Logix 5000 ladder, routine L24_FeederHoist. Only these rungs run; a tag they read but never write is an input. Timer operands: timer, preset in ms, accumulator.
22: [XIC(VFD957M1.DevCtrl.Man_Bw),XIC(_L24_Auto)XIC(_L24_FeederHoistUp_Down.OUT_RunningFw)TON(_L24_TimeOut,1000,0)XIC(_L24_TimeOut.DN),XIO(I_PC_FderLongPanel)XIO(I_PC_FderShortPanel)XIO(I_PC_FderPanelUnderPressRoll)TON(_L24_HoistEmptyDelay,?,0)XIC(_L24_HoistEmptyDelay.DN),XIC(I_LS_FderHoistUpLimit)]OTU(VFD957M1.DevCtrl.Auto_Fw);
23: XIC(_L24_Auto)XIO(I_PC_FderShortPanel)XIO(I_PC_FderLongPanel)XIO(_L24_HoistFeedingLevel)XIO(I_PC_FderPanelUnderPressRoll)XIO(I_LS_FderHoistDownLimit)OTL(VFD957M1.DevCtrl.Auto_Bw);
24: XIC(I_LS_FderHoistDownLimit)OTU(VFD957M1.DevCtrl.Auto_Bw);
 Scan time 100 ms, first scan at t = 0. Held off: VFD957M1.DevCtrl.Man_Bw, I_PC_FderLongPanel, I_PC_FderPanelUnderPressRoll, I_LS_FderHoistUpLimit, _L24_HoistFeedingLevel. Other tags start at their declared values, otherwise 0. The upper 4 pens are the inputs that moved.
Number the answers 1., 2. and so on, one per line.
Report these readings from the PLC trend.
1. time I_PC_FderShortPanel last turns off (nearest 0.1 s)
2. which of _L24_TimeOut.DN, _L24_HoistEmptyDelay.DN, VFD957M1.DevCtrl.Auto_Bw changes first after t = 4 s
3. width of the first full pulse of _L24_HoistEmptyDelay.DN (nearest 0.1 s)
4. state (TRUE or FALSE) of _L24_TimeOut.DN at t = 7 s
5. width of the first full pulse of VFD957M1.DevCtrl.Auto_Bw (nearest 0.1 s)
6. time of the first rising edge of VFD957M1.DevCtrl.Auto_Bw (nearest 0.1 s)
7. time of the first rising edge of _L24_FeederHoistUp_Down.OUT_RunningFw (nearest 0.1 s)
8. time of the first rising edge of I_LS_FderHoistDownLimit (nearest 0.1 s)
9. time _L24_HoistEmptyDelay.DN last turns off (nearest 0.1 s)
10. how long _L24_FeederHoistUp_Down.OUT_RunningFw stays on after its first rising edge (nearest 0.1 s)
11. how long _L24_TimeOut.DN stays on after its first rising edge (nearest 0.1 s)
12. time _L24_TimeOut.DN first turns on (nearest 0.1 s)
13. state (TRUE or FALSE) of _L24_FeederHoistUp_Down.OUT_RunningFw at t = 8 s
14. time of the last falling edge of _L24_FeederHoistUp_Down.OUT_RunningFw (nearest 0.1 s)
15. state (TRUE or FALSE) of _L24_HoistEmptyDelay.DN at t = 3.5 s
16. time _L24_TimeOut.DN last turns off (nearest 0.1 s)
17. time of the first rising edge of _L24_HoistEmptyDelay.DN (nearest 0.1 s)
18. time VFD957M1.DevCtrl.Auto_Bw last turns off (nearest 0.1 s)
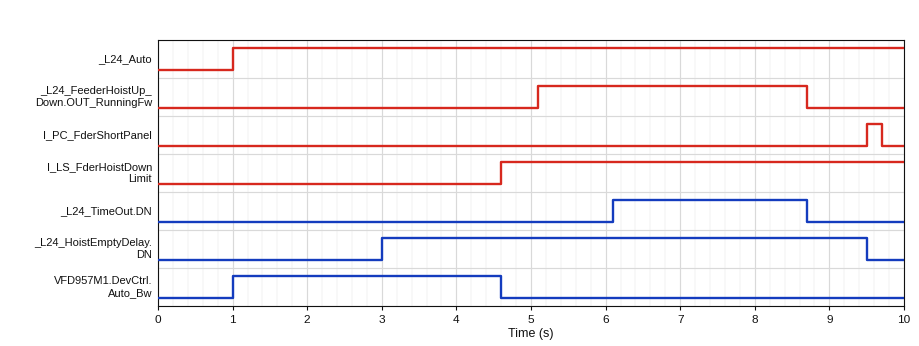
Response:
1. 9.7 s
2. VFD957M1.DevCtrl.Auto_Bw
3. 6.5 s
4. TRUE
5. 3.6 s
6. 1.0 s
7. 5.1 s
8. 4.6 s
9. 9.5 s
10. 3.6 s
11. 2.6 s
12. 6.1 s
13. TRUE
14. 8.7 s
15. TRUE
16. 8.7 s
17. 3.0 s
18. 4.6 s
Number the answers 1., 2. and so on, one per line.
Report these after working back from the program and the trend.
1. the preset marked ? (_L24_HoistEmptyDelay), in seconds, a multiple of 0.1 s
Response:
1. 3.0 s
